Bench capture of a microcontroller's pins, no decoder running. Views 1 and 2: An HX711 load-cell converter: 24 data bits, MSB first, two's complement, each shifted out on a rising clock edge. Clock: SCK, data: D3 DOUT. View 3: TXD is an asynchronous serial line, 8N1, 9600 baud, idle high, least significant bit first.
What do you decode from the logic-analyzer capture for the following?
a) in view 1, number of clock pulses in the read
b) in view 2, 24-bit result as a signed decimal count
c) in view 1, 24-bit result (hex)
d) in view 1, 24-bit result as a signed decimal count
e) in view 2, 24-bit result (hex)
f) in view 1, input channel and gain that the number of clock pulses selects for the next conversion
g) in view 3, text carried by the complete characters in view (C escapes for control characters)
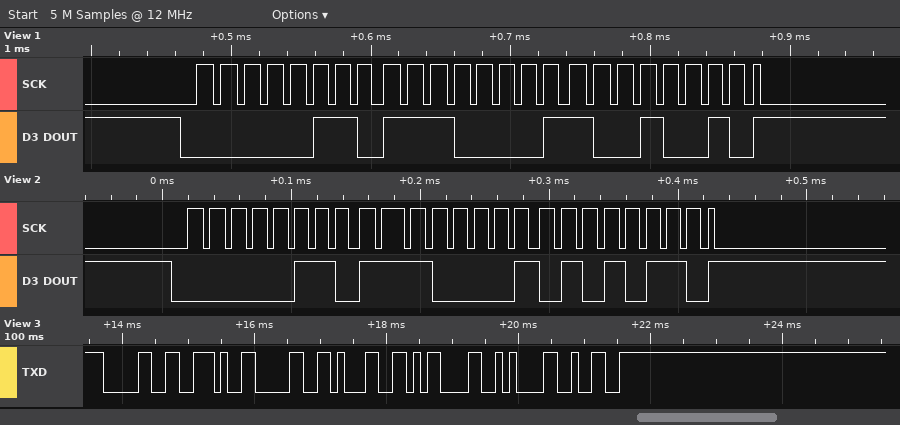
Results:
25
450902
0x06E192
450962
0x06E156
channel A, gain 128
"0.01\r\n2"
